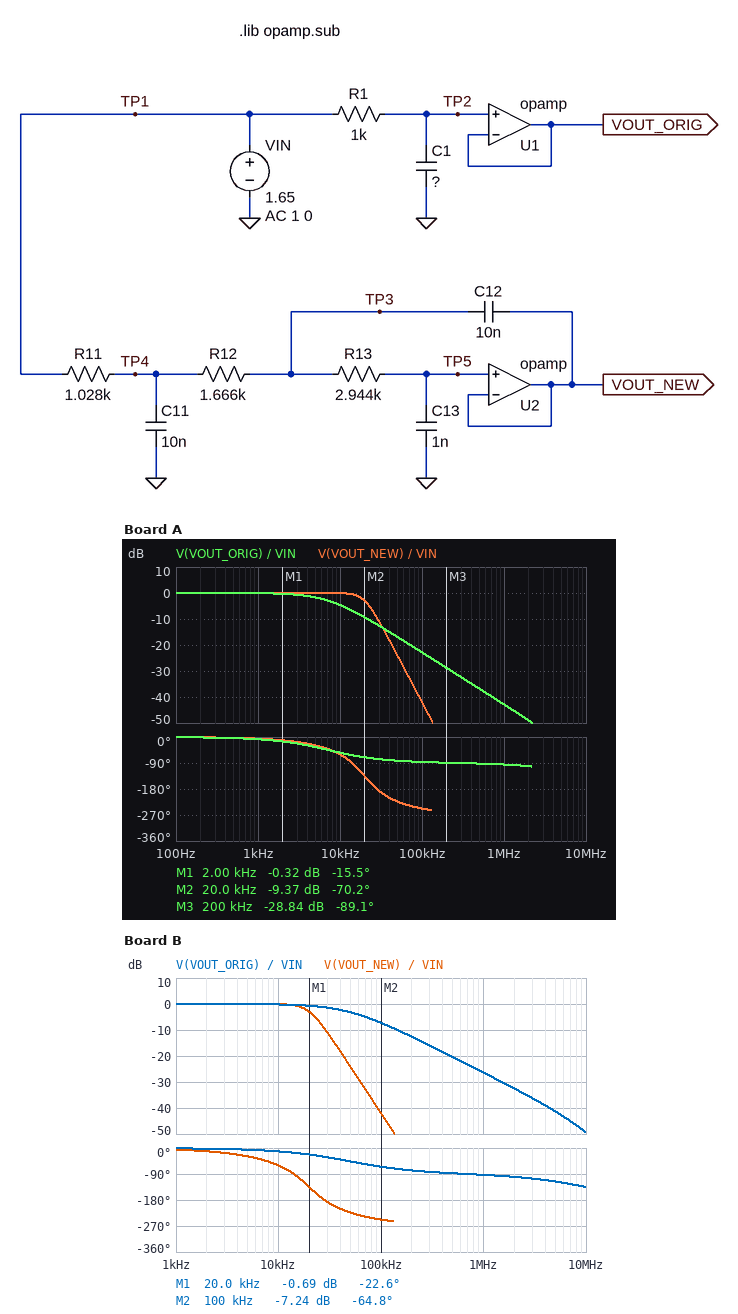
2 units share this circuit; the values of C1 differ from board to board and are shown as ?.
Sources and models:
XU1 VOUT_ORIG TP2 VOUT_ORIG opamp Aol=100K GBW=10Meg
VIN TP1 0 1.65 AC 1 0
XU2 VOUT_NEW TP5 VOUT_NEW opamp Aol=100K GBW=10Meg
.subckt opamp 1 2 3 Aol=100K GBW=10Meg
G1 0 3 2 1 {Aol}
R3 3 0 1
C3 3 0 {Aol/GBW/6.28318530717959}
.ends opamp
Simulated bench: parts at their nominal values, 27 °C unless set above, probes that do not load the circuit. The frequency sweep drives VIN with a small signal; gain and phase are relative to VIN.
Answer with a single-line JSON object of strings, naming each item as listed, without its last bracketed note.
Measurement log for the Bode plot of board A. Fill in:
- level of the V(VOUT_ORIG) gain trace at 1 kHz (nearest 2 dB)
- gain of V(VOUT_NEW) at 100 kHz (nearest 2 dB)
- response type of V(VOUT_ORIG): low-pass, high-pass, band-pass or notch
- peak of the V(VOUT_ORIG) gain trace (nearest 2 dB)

{"level of the V(VOUT_ORIG) gain trace at 1 kHz": "0 dB", "gain of V(VOUT_NEW) at 100 kHz": "-42 dB", "response type of V(VOUT_ORIG): low-pass, high-pass, band-pass or notch": "low-pass", "peak of the V(VOUT_ORIG) gain trace": "0 dB"}
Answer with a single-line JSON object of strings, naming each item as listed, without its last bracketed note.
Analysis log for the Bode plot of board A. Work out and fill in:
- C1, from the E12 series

{"C1, from the E12 series": "22 nF"}
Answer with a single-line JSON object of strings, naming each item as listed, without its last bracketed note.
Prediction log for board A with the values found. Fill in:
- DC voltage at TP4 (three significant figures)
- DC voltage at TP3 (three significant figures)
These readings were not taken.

{"DC voltage at TP4": "1.65 V", "DC voltage at TP3": "1.65 V"}
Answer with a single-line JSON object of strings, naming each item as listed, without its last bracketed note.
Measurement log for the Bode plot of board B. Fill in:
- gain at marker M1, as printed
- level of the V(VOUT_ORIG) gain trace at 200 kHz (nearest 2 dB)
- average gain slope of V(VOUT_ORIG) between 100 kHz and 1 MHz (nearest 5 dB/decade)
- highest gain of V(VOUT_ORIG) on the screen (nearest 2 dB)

{"gain at marker M1, as printed": "-0.69 dB", "level of the V(VOUT_ORIG) gain trace at 200 kHz": "-12 dB", "average gain slope of V(VOUT_ORIG) between 100 kHz and 1 MHz": "-20 dB/decade", "highest gain of V(VOUT_ORIG) on the screen": "0 dB"}
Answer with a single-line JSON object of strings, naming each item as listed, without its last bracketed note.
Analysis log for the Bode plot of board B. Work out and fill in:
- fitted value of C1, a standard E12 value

{"fitted value of C1, a standard E12 value": "3.3 nF"}
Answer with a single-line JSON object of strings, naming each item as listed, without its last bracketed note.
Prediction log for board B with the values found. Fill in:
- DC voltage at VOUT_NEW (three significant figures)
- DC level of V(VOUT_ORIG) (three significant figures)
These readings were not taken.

{"DC voltage at VOUT_NEW": "1.65 V", "DC level of V(VOUT_ORIG)": "1.65 V"}
